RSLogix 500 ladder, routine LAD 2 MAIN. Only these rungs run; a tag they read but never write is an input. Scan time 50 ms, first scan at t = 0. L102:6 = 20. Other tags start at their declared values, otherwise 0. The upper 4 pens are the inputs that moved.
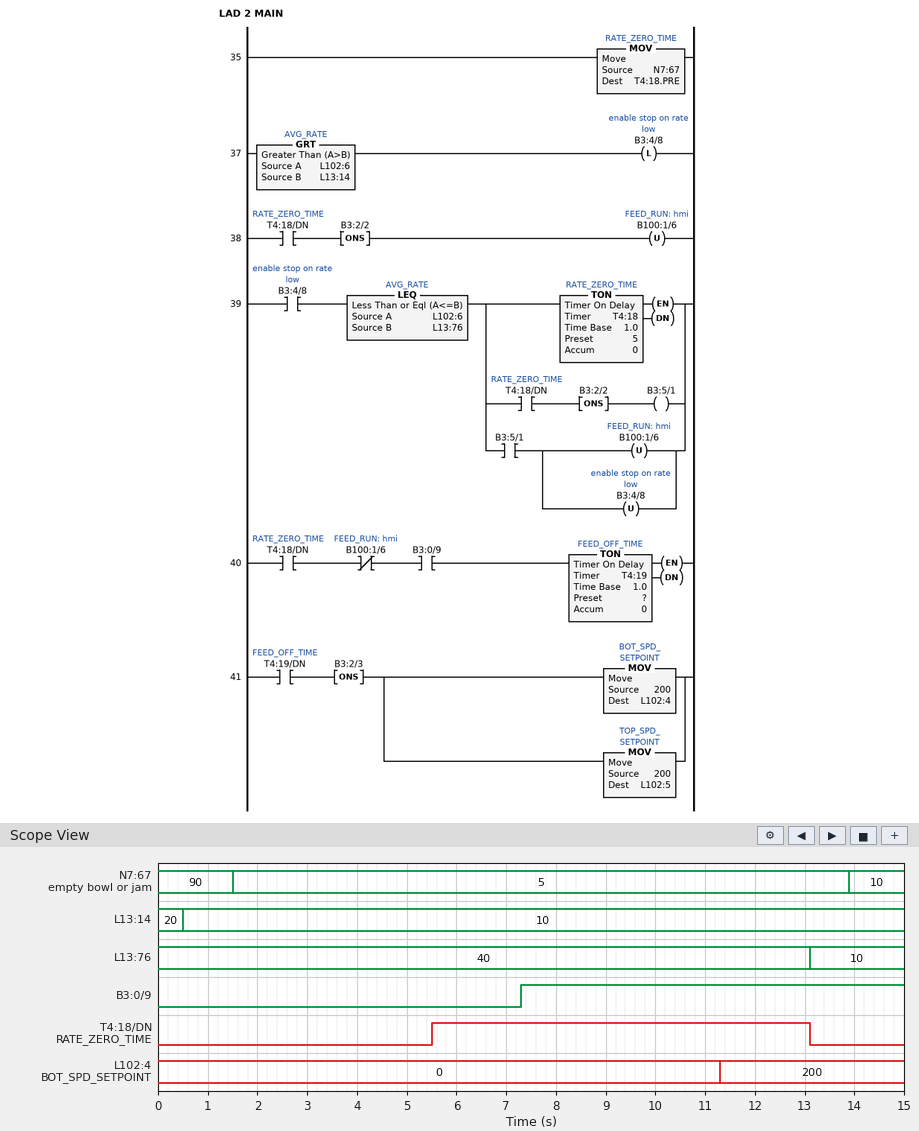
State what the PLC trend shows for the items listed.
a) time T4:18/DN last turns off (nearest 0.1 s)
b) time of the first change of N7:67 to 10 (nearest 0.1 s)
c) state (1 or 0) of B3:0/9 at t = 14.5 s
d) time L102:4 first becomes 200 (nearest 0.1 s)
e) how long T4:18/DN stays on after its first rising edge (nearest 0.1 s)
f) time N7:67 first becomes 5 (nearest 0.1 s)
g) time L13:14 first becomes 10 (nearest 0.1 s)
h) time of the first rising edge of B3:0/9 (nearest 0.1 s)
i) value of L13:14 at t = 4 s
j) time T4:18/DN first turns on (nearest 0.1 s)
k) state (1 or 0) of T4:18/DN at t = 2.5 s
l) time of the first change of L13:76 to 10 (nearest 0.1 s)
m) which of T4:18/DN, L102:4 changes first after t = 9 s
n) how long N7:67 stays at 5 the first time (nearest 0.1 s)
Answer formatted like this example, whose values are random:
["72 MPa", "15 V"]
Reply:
["13.1 s", "13.9 s", "1", "11.3 s", "7.6 s", "1.5 s", "0.5 s", "7.3 s", "10", "5.5 s", "0", "13.1 s", "L102:4", "12.4 s"]
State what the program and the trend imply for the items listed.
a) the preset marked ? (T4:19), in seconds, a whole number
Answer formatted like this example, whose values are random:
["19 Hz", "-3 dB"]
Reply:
["4 s"]
